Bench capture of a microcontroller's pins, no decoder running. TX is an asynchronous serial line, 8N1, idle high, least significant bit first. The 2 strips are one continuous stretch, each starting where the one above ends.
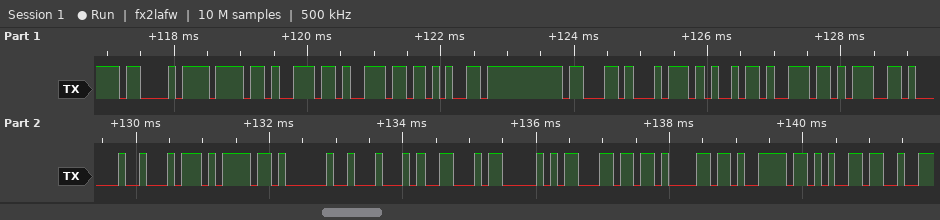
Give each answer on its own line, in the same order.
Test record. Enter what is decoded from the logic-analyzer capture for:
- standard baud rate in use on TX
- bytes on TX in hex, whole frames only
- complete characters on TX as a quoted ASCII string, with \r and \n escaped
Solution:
9600 baud
43 6F 6E 6E 65 63 74 69 6E 67 20 74 6F 20 44 46 50 6C 61 79 65
"Connecting to DFPlaye"
